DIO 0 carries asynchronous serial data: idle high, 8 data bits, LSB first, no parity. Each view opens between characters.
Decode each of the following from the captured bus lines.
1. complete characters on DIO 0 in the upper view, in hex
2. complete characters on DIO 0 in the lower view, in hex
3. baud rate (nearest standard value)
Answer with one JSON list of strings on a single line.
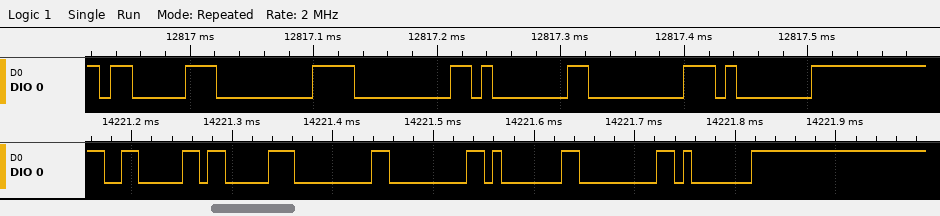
["83, 00, 00, 01, 00, 01", "06, 83, 00, 00, 01, 00, 01", "115200 baud"]
